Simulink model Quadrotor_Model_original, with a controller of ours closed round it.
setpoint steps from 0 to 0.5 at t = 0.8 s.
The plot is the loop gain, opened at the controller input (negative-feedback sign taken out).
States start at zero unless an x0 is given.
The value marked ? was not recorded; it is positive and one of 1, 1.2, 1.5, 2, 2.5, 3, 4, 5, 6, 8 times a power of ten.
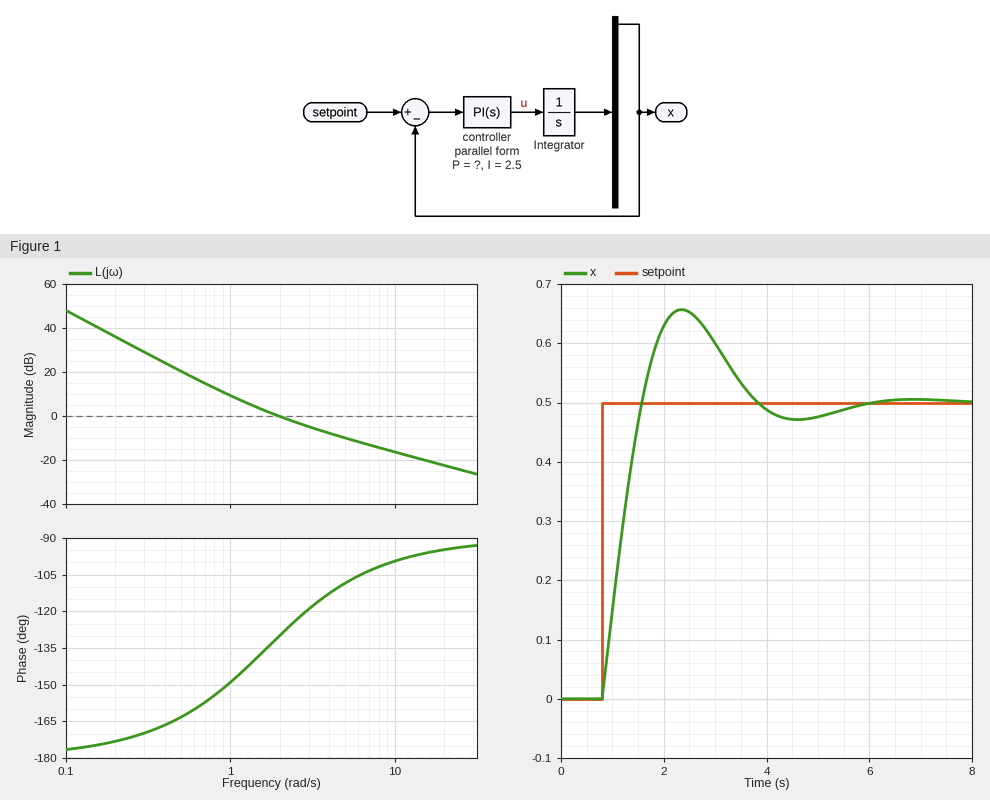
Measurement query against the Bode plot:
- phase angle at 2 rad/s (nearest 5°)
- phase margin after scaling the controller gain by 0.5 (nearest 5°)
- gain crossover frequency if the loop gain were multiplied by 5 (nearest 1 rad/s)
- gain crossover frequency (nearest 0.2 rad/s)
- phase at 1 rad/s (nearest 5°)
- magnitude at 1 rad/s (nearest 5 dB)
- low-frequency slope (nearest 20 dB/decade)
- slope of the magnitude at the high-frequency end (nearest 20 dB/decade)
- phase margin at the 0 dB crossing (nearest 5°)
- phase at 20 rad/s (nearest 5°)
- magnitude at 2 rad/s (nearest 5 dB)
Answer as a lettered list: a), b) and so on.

a) -130°
b) 35°
c) 8 rad/s
d) 2.0 rad/s
e) -150°
f) 10 dB
g) -40 dB/decade
h) -20 dB/decade
i) 50°
j) -95°
k) 0 dB
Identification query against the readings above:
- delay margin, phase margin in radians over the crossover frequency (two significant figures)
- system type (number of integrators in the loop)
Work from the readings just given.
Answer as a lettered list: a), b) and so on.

a) 0.44 s
b) 2
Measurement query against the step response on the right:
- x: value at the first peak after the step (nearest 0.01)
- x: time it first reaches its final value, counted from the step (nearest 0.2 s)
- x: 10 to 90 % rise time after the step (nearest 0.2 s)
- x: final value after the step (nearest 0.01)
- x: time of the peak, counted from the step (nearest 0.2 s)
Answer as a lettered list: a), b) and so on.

a) 0.66
b) 0.8 s
c) 0.6 s
d) 0.50
e) 1.6 s
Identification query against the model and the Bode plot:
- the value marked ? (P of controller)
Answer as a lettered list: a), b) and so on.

a) 1.5
